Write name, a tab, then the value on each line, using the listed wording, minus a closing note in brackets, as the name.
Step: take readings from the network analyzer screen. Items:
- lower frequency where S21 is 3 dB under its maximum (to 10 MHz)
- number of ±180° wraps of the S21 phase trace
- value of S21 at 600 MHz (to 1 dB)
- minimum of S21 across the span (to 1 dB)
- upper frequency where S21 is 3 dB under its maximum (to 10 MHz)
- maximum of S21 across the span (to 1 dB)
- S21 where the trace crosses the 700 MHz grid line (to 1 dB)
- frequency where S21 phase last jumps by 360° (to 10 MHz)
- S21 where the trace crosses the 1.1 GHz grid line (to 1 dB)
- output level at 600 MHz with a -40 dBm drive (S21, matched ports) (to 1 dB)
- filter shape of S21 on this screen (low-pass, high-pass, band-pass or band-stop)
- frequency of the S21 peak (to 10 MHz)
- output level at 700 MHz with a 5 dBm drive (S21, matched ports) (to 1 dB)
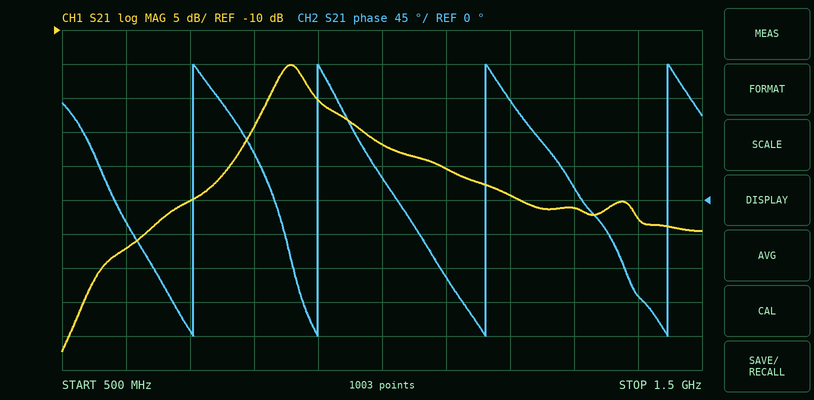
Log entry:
lower frequency where S21 is 3 dB under its maximum	830 MHz
number of ±180° wraps of the S21 phase trace	4
value of S21 at 600 MHz	-42 dB
minimum of S21 across the span	-57 dB
upper frequency where S21 is 3 dB under its maximum	880 MHz
maximum of S21 across the span	-15 dB
S21 where the trace crosses the 700 MHz grid line	-35 dB
frequency where S21 phase last jumps by 360°	1.45 GHz
S21 where the trace crosses the 1.1 GHz grid line	-30 dB
output level at 600 MHz with a -40 dBm drive (S21, matched ports)	-82 dBm
filter shape of S21 on this screen	band-pass
frequency of the S21 peak	860 MHz
output level at 700 MHz with a 5 dBm drive (S21, matched ports)	-30 dBm
